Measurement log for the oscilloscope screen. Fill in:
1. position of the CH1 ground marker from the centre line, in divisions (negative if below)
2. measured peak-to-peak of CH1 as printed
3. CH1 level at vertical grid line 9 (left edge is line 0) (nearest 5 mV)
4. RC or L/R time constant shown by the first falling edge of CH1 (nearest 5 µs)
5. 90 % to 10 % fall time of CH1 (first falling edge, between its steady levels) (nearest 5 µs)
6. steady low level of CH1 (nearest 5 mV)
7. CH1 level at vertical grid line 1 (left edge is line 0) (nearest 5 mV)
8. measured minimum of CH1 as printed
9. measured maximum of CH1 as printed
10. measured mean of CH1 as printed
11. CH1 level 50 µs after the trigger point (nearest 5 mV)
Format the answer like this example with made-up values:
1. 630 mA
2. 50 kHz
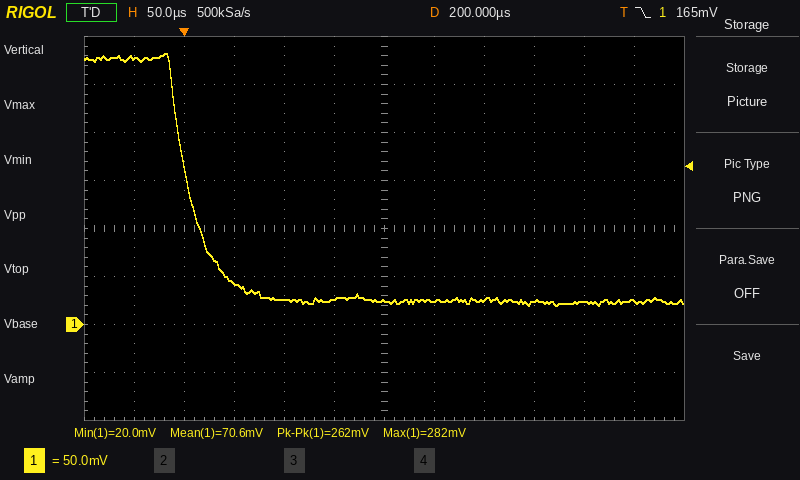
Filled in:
1. -2.0 div
2. 262 mV
3. 25 mV
4. 25 µs
5. 55 µs
6. 25 mV
7. 280 mV
8. 20.0 mV
9. 282 mV
10. 70.6 mV
11. 45 mV
